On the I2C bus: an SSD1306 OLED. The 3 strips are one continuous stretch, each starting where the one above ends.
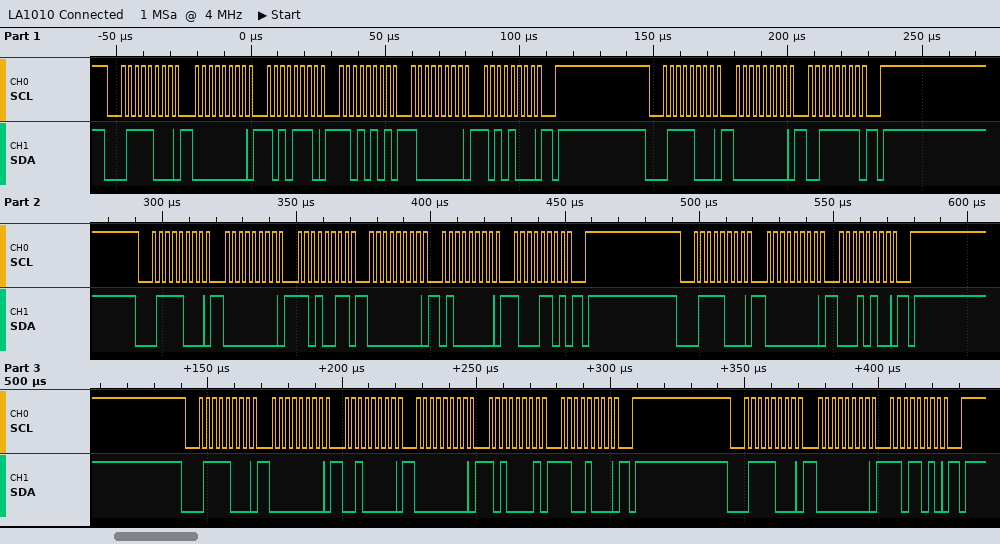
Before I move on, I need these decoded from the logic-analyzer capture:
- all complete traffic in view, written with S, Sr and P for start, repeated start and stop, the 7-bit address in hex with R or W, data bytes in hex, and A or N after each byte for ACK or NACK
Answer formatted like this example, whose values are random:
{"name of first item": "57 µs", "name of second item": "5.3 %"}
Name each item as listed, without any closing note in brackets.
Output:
{"all complete traffic in view, written with S, Sr and P for start, repeated start and stop, the 7-bit address in hex with R or W, data bytes in hex, and A or N after each byte for ACK or NACK": "S 3CW A 00 A AE A D5 A 80 A A8 A P S 3CW A 00 A 3F A P S 3CW A 00 A D3 A 00 A 40 A 8D A P S 3CW A 00 A 14 A P S 3CW A 00 A 20 A 00 A A1 A C8 A P S 3CW A 00 A DA A P"}
